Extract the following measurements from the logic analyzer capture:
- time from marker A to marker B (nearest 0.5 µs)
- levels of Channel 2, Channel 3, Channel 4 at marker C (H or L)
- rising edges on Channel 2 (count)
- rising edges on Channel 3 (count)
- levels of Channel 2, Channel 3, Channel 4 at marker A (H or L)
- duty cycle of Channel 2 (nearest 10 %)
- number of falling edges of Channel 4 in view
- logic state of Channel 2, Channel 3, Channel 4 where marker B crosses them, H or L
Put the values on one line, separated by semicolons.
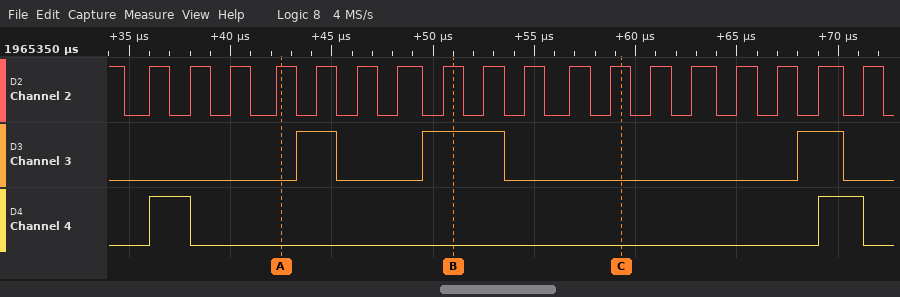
8.5 µs; Channel 2=H, Channel 3=L, Channel 4=L; 18; 3; Channel 2=H, Channel 3=L, Channel 4=L; 50 %; 2; Channel 2=H, Channel 3=H, Channel 4=L
